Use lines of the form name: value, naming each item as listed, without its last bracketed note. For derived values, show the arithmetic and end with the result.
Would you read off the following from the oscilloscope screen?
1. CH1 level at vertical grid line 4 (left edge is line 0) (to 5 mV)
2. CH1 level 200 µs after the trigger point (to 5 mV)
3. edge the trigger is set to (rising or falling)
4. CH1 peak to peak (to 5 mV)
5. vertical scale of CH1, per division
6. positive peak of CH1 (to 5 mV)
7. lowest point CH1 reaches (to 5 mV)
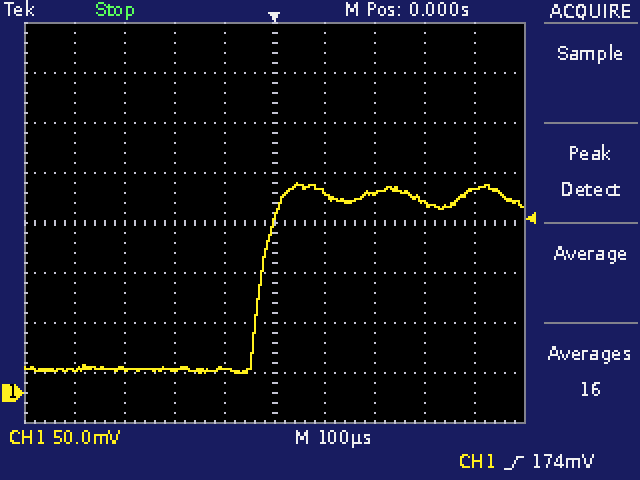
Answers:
CH1 level at vertical grid line 4 (left edge is line 0): 25 mV
CH1 level 200 µs after the trigger point: 200 mV
edge the trigger is set to: rising
CH1 peak to peak: 210 mV − (20 mV) = 190 mV
vertical scale of CH1, per division: 50 mV
positive peak of CH1: 210 mV
lowest point CH1 reaches: 20 mV
